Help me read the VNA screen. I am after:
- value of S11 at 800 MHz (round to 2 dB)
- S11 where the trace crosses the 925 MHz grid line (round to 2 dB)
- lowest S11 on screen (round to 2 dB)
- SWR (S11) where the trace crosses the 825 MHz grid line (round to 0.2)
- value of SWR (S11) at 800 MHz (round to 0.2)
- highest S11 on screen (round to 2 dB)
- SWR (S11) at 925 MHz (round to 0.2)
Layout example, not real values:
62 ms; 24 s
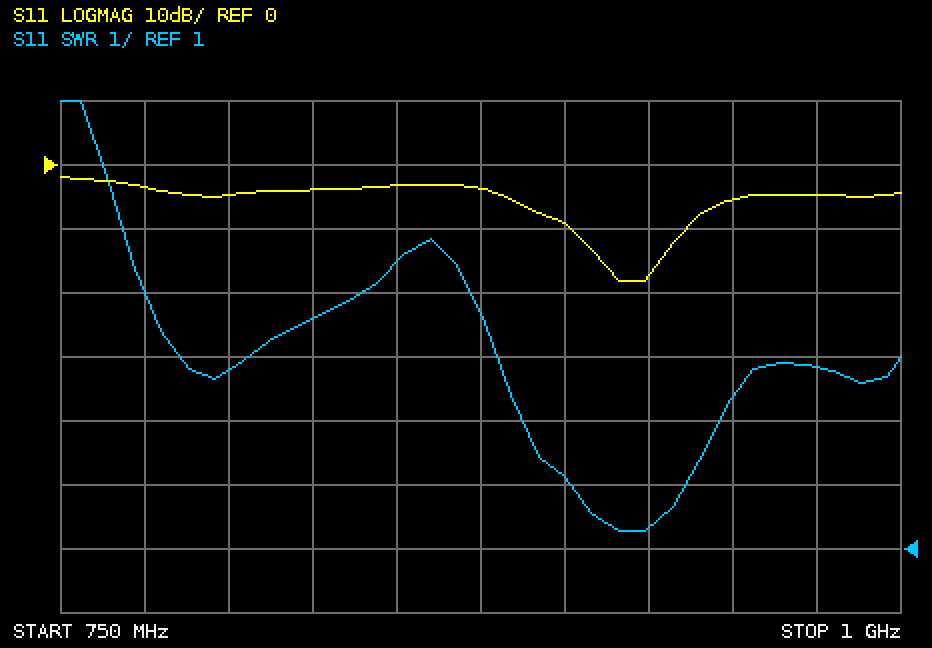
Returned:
-4 dB; -18 dB; -18 dB; 4.6; 3.8; -2 dB; 1.4
